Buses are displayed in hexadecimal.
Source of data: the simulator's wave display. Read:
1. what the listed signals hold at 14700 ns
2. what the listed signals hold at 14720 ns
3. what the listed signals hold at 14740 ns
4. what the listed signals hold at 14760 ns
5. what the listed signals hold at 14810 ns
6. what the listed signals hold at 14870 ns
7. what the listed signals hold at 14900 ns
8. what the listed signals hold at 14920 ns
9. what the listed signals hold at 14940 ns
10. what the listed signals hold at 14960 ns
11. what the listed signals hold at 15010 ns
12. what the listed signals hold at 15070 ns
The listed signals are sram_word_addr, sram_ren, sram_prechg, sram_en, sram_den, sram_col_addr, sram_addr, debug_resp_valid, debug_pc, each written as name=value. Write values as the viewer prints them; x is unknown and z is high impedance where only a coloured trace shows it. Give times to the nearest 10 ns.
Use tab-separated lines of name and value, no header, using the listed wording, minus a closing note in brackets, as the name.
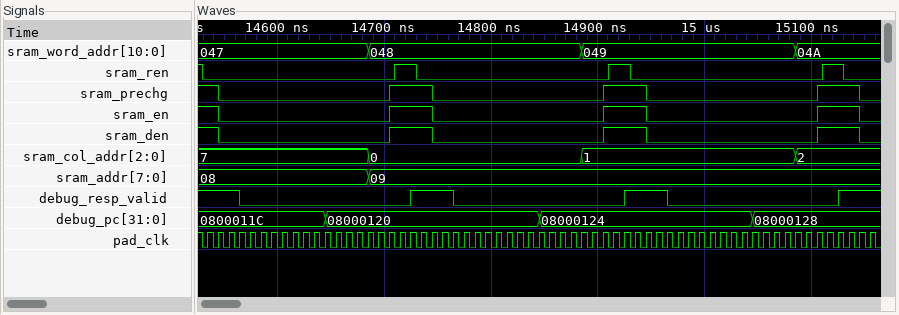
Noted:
what the listed signals hold at 14700 ns	sram_word_addr=048, sram_ren=0, sram_prechg=0, sram_en=0, sram_den=0, sram_col_addr=0, sram_addr=09, debug_resp_valid=0, debug_pc=08000120
what the listed signals hold at 14720 ns	sram_word_addr=048, sram_ren=1, sram_prechg=1, sram_en=1, sram_den=1, sram_col_addr=0, sram_addr=09, debug_resp_valid=0, debug_pc=08000120
what the listed signals hold at 14740 ns	sram_word_addr=048, sram_ren=0, sram_prechg=1, sram_en=1, sram_den=1, sram_col_addr=0, sram_addr=09, debug_resp_valid=1, debug_pc=08000120
what the listed signals hold at 14760 ns	sram_word_addr=048, sram_ren=0, sram_prechg=0, sram_en=0, sram_den=0, sram_col_addr=0, sram_addr=09, debug_resp_valid=1, debug_pc=08000120
what the listed signals hold at 14810 ns	sram_word_addr=048, sram_ren=0, sram_prechg=0, sram_en=0, sram_den=0, sram_col_addr=0, sram_addr=09, debug_resp_valid=0, debug_pc=08000120
what the listed signals hold at 14870 ns	sram_word_addr=048, sram_ren=0, sram_prechg=0, sram_en=0, sram_den=0, sram_col_addr=0, sram_addr=09, debug_resp_valid=0, debug_pc=08000124
what the listed signals hold at 14900 ns	sram_word_addr=049, sram_ren=0, sram_prechg=0, sram_en=0, sram_den=0, sram_col_addr=1, sram_addr=09, debug_resp_valid=0, debug_pc=08000124
what the listed signals hold at 14920 ns	sram_word_addr=049, sram_ren=1, sram_prechg=1, sram_en=1, sram_den=1, sram_col_addr=1, sram_addr=09, debug_resp_valid=0, debug_pc=08000124
what the listed signals hold at 14940 ns	sram_word_addr=049, sram_ren=0, sram_prechg=1, sram_en=1, sram_den=1, sram_col_addr=1, sram_addr=09, debug_resp_valid=1, debug_pc=08000124
what the listed signals hold at 14960 ns	sram_word_addr=049, sram_ren=0, sram_prechg=0, sram_en=0, sram_den=0, sram_col_addr=1, sram_addr=09, debug_resp_valid=1, debug_pc=08000124
what the listed signals hold at 15010 ns	sram_word_addr=049, sram_ren=0, sram_prechg=0, sram_en=0, sram_den=0, sram_col_addr=1, sram_addr=09, debug_resp_valid=0, debug_pc=08000124
what the listed signals hold at 15070 ns	sram_word_addr=049, sram_ren=0, sram_prechg=0, sram_en=0, sram_den=0, sram_col_addr=1, sram_addr=09, debug_resp_valid=0, debug_pc=08000128
